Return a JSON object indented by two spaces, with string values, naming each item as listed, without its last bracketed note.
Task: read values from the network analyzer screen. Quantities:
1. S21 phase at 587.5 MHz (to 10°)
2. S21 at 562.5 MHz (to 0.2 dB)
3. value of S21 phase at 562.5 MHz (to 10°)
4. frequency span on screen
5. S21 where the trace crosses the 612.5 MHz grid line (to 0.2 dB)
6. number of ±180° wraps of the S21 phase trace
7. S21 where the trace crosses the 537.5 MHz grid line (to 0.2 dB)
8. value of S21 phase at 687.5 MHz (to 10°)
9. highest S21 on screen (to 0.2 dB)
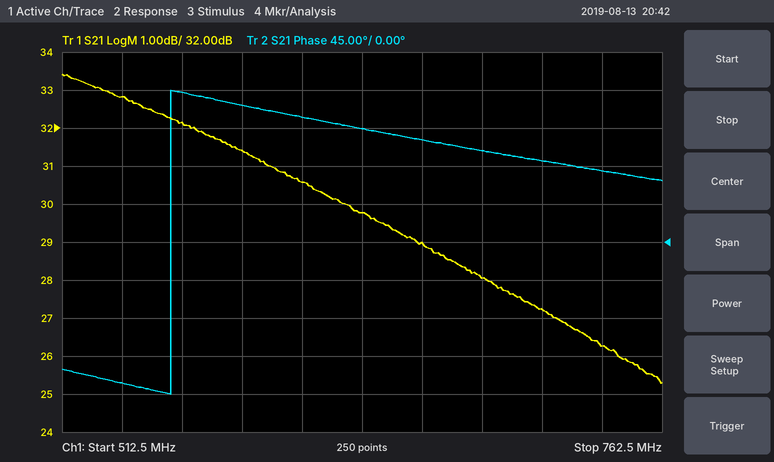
{
  "S21 phase at 587.5 MHz": "160°",
  "S21 at 562.5 MHz": "32.2 dB",
  "value of S21 phase at 562.5 MHz": "180°",
  "frequency span on screen": "250 MHz",
  "S21 where the trace crosses the 612.5 MHz grid line": "30.6 dB",
  "number of ±180° wraps of the S21 phase trace": "1",
  "S21 where the trace crosses the 537.5 MHz grid line": "32.8 dB",
  "value of S21 phase at 687.5 MHz": "110°",
  "highest S21 on screen": "33.4 dB"
}
